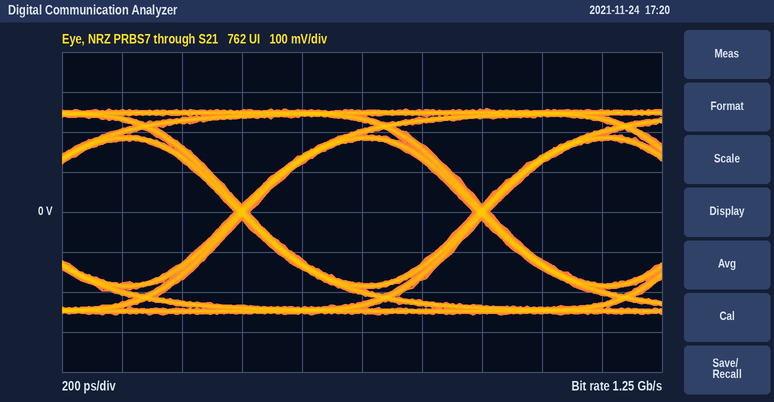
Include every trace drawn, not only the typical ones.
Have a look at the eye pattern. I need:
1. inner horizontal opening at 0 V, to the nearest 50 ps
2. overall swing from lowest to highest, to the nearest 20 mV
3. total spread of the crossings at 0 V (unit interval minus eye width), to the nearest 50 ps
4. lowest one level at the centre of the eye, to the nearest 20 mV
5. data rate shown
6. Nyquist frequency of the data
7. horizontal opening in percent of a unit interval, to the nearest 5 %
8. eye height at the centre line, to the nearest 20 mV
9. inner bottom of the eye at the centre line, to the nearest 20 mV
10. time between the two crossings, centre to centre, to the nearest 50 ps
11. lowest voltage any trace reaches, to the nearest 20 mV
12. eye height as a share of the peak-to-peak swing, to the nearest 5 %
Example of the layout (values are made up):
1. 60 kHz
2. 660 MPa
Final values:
1. 750 ps
2. 520 mV
3. 50 ps
4. 180 mV
5. 1.25 Gb/s
6. 625 MHz
7. 95 %
8. 360 mV
9. -180 mV
10. 800 ps
11. -260 mV
12. 70 %
